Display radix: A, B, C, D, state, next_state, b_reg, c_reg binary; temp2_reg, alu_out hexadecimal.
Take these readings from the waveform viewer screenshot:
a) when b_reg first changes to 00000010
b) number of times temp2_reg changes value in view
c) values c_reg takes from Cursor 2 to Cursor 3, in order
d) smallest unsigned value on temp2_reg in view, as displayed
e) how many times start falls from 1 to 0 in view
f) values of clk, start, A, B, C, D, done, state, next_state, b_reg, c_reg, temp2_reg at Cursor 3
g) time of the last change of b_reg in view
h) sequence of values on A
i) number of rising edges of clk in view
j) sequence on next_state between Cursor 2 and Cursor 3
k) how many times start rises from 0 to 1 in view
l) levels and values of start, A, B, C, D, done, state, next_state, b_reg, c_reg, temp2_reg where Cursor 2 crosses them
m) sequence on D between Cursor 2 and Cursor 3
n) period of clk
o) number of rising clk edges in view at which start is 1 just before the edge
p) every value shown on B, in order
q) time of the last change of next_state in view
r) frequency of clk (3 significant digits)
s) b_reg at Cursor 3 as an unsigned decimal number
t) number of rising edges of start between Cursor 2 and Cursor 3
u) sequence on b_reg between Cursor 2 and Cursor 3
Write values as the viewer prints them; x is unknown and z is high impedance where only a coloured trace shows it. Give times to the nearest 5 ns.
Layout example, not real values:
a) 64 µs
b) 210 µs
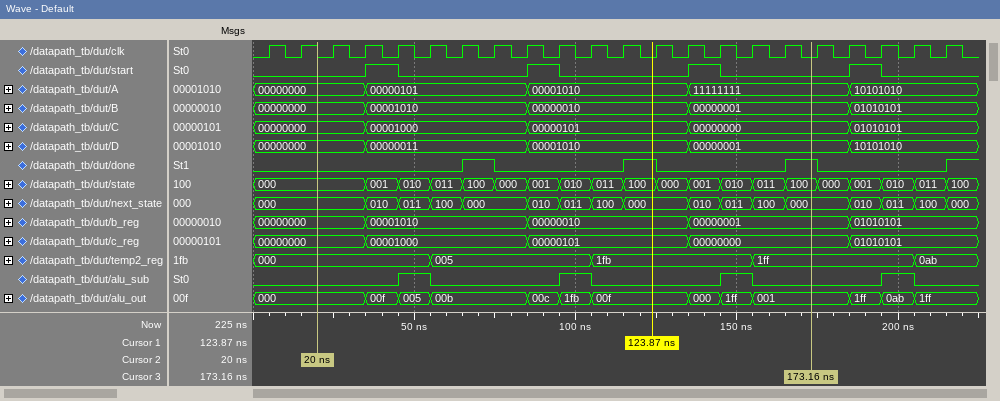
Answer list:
a) 85 ns
b) 4
c) 00000000, 00001000, 00000101, 00000000
d) 000
e) 4
f) clk=0, start=0, A=11111111, B=00000001, C=00000000, D=00000001, done=1, state=100, next_state=000, b_reg=00000001, c_reg=00000000, temp2_reg=1ff
g) 185 ns
h) 00000000, 00000101, 00001010, 11111111, 10101010
i) 22
j) 000, 010, 011, 100, 000, 010, 011, 100, 000, 010, 011, 100, 000
k) 4
l) start=0, A=00000000, B=00000000, C=00000000, D=00000000, done=0, state=000, next_state=000, b_reg=00000000, c_reg=00000000, temp2_reg=000
m) 00000000, 00000011, 00001010, 00000001
n) 10 ns
o) 4
p) 00000000, 00001010, 00000010, 00000001, 01010101
q) 215 ns
r) 100 MHz
s) 1
t) 3
u) 00000000, 00001010, 00000010, 00000001
